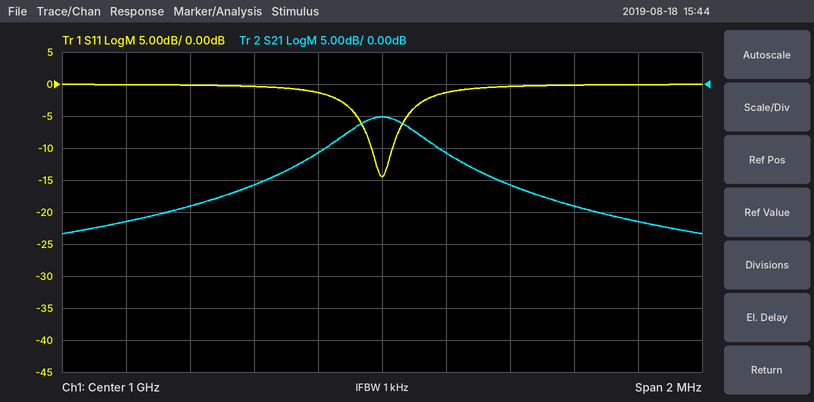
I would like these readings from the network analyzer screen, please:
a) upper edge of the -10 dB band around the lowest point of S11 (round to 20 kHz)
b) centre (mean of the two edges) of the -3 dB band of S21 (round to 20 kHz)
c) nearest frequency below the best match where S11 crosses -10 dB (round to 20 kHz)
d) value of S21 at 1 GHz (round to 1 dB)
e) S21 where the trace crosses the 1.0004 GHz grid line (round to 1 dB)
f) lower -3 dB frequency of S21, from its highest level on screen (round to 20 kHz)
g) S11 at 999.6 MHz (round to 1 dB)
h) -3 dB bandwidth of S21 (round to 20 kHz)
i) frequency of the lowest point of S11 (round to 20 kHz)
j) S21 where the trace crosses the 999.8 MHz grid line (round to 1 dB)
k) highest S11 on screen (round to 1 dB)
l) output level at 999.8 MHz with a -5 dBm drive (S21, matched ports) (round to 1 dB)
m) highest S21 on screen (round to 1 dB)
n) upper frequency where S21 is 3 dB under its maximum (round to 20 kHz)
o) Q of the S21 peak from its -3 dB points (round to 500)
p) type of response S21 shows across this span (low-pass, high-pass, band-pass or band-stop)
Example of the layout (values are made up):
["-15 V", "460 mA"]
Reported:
["1.00004 GHz", "1.00000 GHz", "999.96 MHz", "-5 dB", "-16 dB", "999.88 MHz", "0 dB", "240 kHz", "1.00000 GHz", "-11 dB", "0 dB", "-16 dBm", "-5 dB", "1.00012 GHz", "4000", "band-pass"]
